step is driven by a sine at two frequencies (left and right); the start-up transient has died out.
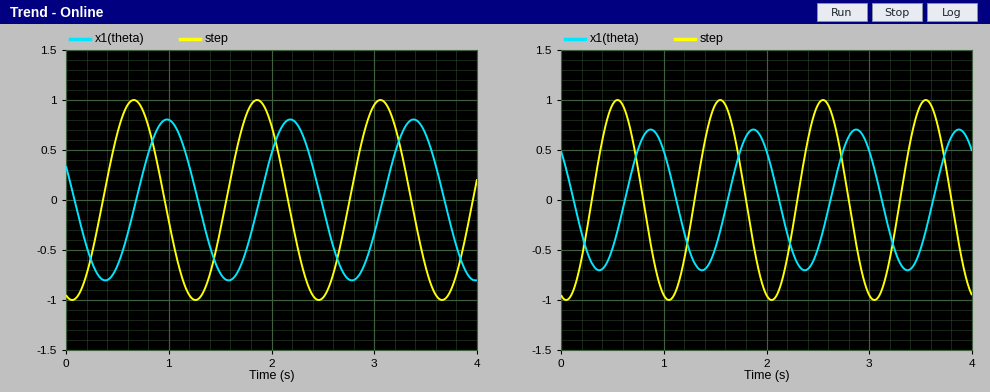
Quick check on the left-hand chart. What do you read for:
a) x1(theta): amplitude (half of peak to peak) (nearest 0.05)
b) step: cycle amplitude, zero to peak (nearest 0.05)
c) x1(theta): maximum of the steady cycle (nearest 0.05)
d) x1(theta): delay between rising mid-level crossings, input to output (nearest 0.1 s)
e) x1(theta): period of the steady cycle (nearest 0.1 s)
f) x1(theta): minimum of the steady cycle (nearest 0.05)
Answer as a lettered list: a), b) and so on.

a) 0.80
b) 1.00
c) 0.80
d) 0.3 s
e) 1.2 s
f) -0.80
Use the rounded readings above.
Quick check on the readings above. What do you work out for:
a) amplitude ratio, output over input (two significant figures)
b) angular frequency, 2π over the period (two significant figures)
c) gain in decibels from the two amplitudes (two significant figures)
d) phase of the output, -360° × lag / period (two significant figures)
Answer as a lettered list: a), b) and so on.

a) 0.80
b) 5.2 rad/s
c) -1.9 dB
d) -90°
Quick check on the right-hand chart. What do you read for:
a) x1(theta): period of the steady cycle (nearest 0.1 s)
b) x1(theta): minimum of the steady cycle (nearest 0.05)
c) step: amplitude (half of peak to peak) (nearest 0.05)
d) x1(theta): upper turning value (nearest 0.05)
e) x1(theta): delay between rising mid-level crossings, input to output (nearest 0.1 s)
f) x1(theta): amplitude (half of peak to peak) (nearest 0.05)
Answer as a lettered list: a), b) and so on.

a) 1.0 s
b) -0.70
c) 1.00
d) 0.70
e) 0.3 s
f) 0.70
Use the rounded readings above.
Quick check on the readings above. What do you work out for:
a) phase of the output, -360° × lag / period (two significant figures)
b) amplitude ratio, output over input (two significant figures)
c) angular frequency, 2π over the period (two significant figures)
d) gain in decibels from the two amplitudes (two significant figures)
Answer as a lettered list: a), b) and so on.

a) -110°
b) 0.70
c) 6.3 rad/s
d) -3.1 dB
